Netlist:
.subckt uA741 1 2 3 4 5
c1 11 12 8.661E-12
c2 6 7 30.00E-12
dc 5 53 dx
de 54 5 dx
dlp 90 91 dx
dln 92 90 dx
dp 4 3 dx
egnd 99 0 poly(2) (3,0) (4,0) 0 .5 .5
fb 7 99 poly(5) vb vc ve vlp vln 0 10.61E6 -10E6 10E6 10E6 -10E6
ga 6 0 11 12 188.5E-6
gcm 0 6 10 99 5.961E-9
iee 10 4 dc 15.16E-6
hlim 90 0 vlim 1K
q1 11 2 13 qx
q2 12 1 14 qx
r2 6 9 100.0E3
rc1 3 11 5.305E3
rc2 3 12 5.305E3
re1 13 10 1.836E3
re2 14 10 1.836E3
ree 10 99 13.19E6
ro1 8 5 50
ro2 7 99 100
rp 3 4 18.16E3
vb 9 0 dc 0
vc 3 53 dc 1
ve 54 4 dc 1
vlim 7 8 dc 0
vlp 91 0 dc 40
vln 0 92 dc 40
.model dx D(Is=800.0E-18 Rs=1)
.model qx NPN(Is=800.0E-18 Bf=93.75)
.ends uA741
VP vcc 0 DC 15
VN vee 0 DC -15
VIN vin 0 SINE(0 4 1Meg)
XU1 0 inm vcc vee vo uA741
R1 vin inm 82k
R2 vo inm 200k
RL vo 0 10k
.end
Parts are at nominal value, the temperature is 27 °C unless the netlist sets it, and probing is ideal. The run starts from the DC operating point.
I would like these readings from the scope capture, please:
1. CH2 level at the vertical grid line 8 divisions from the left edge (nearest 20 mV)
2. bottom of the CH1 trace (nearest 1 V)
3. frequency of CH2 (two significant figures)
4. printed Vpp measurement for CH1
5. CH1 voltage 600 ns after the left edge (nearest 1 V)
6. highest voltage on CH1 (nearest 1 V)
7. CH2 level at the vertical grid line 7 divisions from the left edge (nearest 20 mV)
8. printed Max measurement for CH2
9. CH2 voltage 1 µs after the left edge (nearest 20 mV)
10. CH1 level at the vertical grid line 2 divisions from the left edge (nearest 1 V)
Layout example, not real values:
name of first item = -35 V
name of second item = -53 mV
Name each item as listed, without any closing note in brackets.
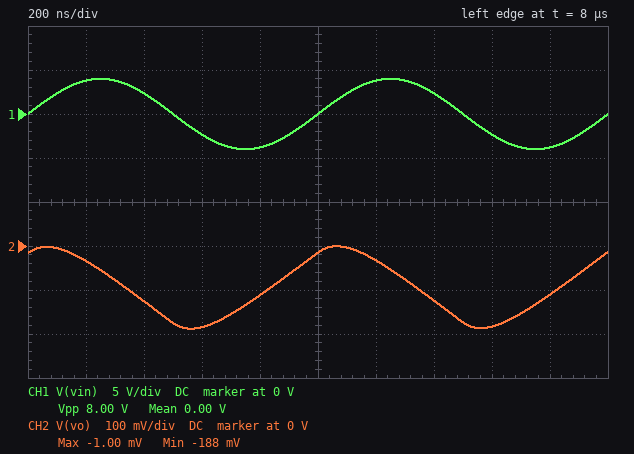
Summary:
CH2 level at the vertical grid line 8 divisions from the left edge = -180 mV
bottom of the CH1 trace = -4 V
frequency of CH2 = 1.0 MHz
printed Vpp measurement for CH1 = 8.00 V
CH1 voltage 600 ns after the left edge = -2 V
highest voltage on CH1 = 4 V
CH2 level at the vertical grid line 7 divisions from the left edge = -120 mV
printed Max measurement for CH2 = -1.00 mV
CH2 voltage 1 µs after the left edge = -20 mV
CH1 level at the vertical grid line 2 divisions from the left edge = 2 V
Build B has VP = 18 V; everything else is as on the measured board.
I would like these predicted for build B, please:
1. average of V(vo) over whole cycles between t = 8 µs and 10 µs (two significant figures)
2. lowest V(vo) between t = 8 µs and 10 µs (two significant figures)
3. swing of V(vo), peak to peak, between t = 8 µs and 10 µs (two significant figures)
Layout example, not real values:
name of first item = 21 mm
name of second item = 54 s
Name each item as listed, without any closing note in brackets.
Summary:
average of V(vo) over whole cycles between t = 8 µs and 10 µs = -91 mV
lowest V(vo) between t = 8 µs and 10 µs = -180 mV
swing of V(vo), peak to peak, between t = 8 µs and 10 µs = 190 mV
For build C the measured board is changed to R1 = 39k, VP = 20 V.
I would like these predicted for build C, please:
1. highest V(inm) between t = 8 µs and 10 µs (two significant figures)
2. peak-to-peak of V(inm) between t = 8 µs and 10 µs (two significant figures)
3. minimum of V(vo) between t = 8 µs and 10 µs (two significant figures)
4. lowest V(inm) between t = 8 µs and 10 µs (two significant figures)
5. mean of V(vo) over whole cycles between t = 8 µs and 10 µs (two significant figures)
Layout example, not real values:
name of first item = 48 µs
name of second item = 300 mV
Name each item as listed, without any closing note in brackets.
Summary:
highest V(inm) between t = 8 µs and 10 µs = 3.3 V
peak-to-peak of V(inm) between t = 8 µs and 10 µs = 6.7 V
minimum of V(vo) between t = 8 µs and 10 µs = -200 mV
lowest V(inm) between t = 8 µs and 10 µs = -3.4 V
mean of V(vo) over whole cycles between t = 8 µs and 10 µs = -110 mV
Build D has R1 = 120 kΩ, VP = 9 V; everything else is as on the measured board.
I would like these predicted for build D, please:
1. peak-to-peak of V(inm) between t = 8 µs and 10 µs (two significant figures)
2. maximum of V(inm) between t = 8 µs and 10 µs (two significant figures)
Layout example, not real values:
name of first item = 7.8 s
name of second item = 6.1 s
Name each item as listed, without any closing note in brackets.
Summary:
peak-to-peak of V(inm) between t = 8 µs and 10 µs = 5.0 V
maximum of V(inm) between t = 8 µs and 10 µs = 2.5 V
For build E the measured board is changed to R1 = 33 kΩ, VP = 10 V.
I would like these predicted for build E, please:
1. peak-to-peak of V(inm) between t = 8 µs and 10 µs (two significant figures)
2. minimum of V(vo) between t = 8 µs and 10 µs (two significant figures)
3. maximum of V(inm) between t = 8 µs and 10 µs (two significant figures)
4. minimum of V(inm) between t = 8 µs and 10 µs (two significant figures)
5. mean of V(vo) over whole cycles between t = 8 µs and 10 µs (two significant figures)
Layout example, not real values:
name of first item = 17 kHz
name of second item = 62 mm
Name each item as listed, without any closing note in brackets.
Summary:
peak-to-peak of V(inm) between t = 8 µs and 10 µs = 6.9 V
minimum of V(vo) between t = 8 µs and 10 µs = -220 mV
maximum of V(inm) between t = 8 µs and 10 µs = 3.4 V
minimum of V(inm) between t = 8 µs and 10 µs = -3.5 V
mean of V(vo) over whole cycles between t = 8 µs and 10 µs = -120 mV
